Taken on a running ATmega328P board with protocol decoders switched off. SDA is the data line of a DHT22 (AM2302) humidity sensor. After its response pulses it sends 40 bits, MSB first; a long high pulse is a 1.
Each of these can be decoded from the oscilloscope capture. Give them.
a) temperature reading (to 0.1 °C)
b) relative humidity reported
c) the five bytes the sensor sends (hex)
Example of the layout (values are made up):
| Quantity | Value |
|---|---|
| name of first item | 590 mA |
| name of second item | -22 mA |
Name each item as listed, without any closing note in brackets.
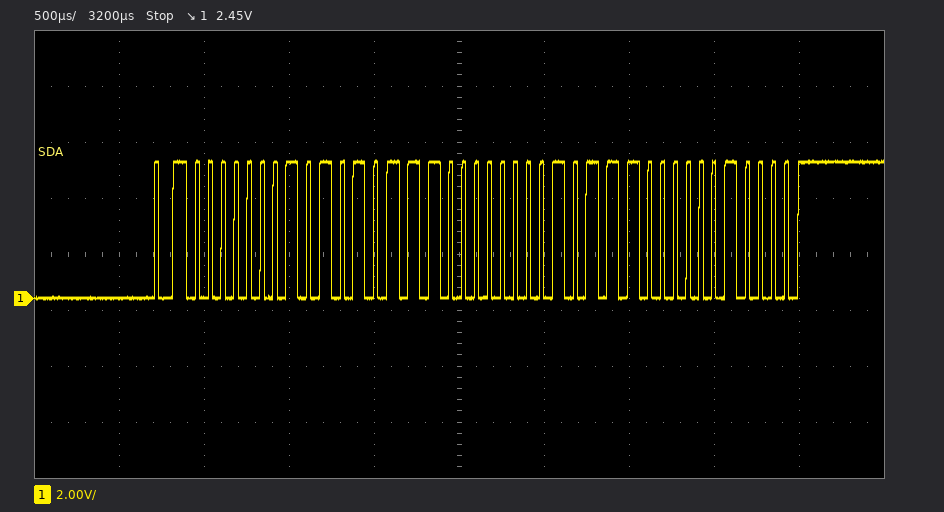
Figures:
| Quantity | Value |
|---|---|
| temperature reading | 18.4 °C |
| relative humidity reported | 34.3 % |
| the five bytes the sensor sends | 01 57 00 B8 10 |
